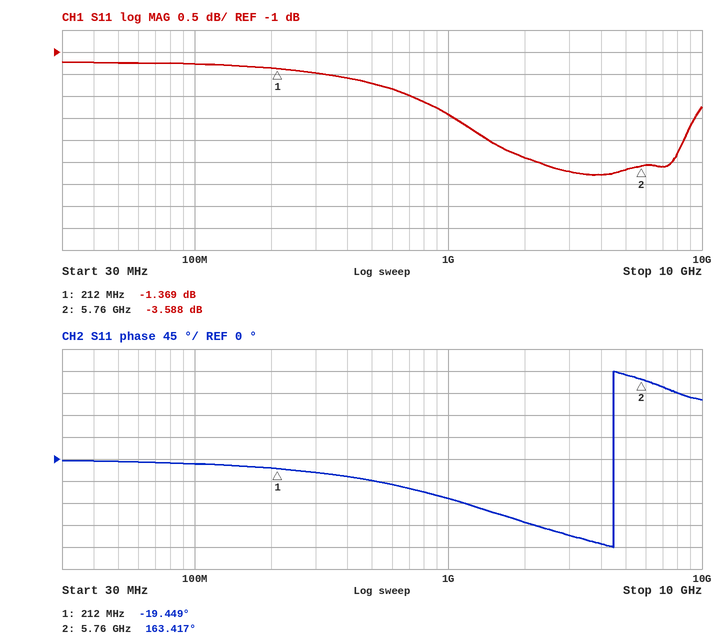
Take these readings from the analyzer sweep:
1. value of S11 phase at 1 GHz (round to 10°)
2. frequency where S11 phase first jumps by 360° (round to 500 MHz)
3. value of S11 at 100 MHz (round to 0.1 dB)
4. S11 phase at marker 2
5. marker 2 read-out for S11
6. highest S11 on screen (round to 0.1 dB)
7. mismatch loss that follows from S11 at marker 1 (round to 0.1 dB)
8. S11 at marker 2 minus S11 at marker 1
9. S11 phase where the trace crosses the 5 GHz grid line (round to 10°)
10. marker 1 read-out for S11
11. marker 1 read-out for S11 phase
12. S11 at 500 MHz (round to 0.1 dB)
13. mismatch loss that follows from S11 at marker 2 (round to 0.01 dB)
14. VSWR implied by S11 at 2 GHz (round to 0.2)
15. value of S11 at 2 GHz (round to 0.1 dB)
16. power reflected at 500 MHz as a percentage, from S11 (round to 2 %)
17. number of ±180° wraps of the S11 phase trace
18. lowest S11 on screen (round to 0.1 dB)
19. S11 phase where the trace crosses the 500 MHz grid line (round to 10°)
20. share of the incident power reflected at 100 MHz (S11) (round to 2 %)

-80°
4.5 GHz
-1.3 dB
163.417°
-3.588 dB
-1.2 dB
5.7 dB
-2.219 dB
170°
-1.369 dB
-19.449°
-1.7 dB
2.50 dB
5.2
-3.4 dB
68 %
1
-3.8 dB
-40°
74 %
